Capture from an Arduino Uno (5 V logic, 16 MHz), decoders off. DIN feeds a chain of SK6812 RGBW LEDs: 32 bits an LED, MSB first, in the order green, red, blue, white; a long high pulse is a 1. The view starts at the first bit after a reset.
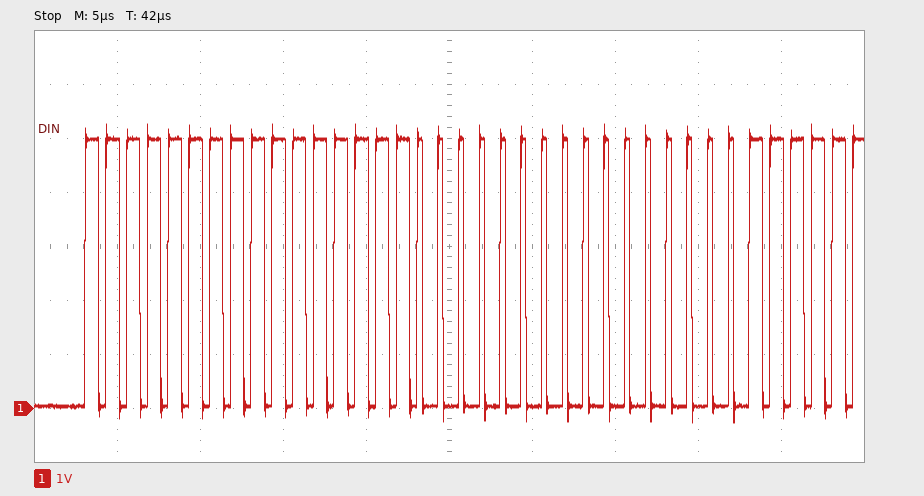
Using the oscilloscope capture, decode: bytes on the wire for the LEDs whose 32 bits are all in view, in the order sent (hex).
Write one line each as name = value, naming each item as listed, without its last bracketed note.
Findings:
bytes on the wire for the LEDs whose 32 bits are all in view, in the order sent = FF FF 00 00
